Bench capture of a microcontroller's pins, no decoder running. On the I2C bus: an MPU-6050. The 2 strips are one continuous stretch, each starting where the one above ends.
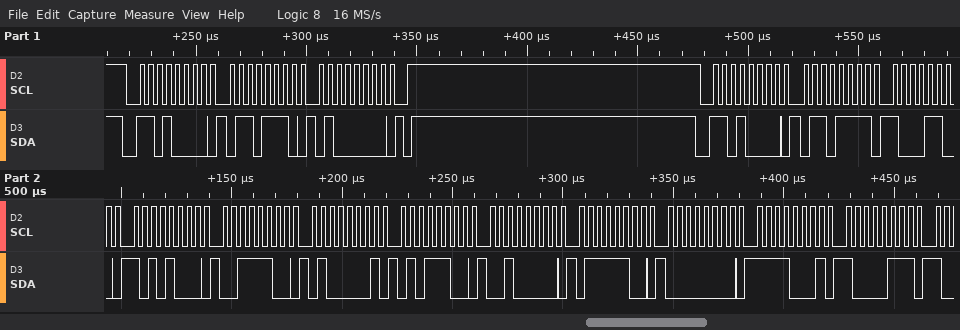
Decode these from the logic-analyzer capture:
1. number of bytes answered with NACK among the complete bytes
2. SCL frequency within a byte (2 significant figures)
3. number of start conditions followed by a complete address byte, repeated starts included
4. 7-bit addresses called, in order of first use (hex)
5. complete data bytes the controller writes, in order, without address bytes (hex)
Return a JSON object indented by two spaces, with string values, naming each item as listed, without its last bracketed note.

{
  "number of bytes answered with NACK among the complete bytes": "0",
  "SCL frequency within a byte": "250 kHz",
  "number of start conditions followed by a complete address byte, repeated starts included": "2",
  "7-bit addresses called, in order of first use": "0x68",
  "complete data bytes the controller writes, in order, without address bytes": "6E 40 6F 8C A8 3C 41 5C 20 7C 00 F1 87"
}
